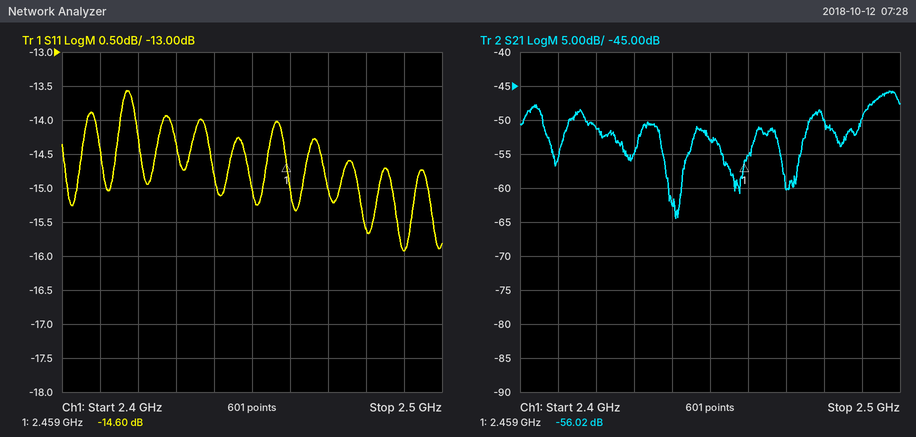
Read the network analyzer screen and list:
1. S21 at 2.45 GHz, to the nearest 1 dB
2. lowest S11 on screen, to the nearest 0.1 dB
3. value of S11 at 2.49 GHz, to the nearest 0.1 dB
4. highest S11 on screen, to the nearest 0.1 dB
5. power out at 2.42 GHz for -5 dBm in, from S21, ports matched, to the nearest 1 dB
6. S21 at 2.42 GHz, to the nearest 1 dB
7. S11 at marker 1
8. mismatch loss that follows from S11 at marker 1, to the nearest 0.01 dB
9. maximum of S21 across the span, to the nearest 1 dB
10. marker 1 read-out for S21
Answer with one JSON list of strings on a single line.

["-53 dB", "-15.9 dB", "-15.9 dB", "-13.6 dB", "-56 dBm", "-51 dB", "-14.60 dB", "0.15 dB", "-46 dB", "-56.02 dB"]
